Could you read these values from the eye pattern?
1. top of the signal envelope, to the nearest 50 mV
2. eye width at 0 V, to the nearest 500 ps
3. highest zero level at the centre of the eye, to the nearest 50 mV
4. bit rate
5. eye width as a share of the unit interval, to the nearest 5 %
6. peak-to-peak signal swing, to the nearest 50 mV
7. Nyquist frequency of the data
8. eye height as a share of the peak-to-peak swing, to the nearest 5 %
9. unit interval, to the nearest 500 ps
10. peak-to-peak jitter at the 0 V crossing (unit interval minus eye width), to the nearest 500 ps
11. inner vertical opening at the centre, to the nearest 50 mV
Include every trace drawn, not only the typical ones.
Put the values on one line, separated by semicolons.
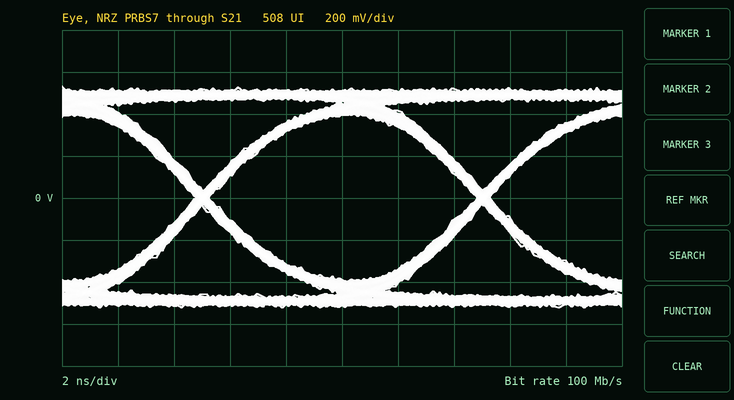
550 mV; 9.5 ns; -400 mV; 100 Mb/s; 95 %; 1.05 V; 50 MHz; 75 %; 10.0 ns; 500 ps; 800 mV
